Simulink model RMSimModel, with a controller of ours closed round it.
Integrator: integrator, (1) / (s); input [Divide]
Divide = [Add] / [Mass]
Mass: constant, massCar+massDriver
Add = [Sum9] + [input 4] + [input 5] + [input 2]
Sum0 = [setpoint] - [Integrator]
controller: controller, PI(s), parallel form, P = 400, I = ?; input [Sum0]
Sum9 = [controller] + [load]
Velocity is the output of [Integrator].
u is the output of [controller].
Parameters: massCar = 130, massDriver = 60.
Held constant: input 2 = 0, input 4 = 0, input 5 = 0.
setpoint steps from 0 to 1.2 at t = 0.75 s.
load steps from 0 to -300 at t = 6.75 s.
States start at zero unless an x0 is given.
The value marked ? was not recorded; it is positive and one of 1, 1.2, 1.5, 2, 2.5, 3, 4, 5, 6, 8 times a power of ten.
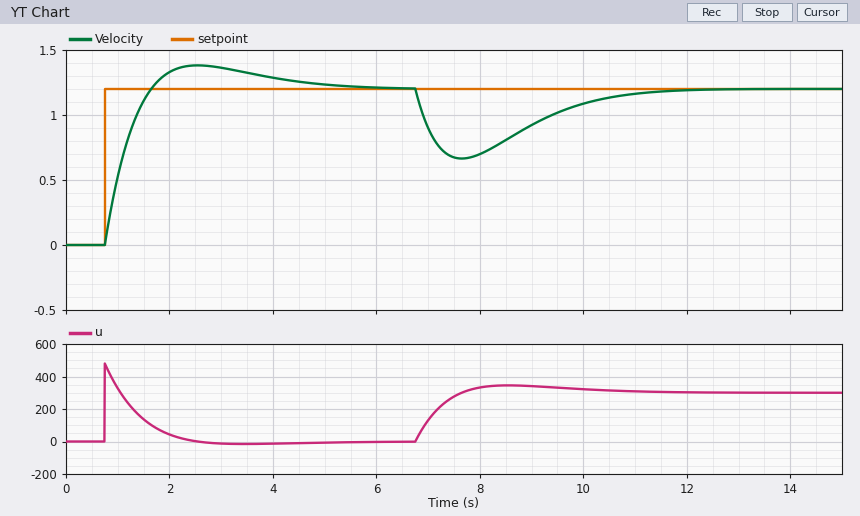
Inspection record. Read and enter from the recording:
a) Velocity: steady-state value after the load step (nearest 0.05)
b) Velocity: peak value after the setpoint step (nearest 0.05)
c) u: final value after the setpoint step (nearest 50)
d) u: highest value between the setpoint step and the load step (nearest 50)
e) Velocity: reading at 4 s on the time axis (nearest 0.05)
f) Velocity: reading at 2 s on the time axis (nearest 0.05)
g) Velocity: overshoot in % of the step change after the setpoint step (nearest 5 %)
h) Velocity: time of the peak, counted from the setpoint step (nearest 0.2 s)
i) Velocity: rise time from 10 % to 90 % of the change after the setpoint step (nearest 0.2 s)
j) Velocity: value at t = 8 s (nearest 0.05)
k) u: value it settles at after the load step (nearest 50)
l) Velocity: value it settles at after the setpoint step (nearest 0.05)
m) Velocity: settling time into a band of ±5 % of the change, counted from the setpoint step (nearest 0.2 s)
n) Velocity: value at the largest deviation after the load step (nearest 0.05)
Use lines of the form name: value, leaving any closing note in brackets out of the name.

Velocity: steady-state value after the load step: 1.20
Velocity: peak value after the setpoint step: 1.40
u: final value after the setpoint step: 0
u: highest value between the setpoint step and the load step: 500
Velocity: reading at 4 s on the time axis: 1.30
Velocity: reading at 2 s on the time axis: 1.35
Velocity: overshoot in % of the step change after the setpoint step: 15 %
Velocity: time of the peak, counted from the setpoint step: 1.8 s
Velocity: rise time from 10 % to 90 % of the change after the setpoint step: 0.6 s
Velocity: value at t = 8 s: 0.70
u: value it settles at after the load step: 300
Velocity: value it settles at after the setpoint step: 1.20
Velocity: settling time into a band of ±5 % of the change, counted from the setpoint step: 3.6 s
Velocity: value at the largest deviation after the load step: 0.65
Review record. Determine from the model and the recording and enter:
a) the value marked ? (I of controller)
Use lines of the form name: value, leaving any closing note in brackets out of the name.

the value marked ?: 250
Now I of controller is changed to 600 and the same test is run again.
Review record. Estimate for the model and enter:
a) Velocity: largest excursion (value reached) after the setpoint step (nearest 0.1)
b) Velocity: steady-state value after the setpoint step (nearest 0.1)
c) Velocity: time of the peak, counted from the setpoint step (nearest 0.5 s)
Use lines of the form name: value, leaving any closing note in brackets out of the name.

Velocity: largest excursion (value reached) after the setpoint step: 1.5
Velocity: steady-state value after the setpoint step: 1.2
Velocity: time of the peak, counted from the setpoint step: 1.5 s
